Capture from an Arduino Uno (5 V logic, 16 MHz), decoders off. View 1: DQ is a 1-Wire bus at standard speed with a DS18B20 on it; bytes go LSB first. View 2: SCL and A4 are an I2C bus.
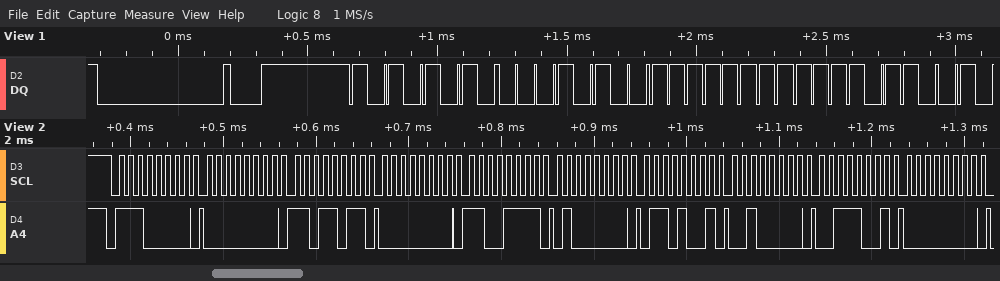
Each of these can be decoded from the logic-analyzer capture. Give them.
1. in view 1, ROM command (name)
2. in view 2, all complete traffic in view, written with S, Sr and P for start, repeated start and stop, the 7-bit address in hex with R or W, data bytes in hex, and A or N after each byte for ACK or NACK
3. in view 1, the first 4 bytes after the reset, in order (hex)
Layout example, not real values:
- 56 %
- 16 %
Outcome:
- Match ROM
- S 70W A 00 A DB A 00 A CF A 40 A 69 A 20 A 39 A 00 A
- 55 28 FF 6F
